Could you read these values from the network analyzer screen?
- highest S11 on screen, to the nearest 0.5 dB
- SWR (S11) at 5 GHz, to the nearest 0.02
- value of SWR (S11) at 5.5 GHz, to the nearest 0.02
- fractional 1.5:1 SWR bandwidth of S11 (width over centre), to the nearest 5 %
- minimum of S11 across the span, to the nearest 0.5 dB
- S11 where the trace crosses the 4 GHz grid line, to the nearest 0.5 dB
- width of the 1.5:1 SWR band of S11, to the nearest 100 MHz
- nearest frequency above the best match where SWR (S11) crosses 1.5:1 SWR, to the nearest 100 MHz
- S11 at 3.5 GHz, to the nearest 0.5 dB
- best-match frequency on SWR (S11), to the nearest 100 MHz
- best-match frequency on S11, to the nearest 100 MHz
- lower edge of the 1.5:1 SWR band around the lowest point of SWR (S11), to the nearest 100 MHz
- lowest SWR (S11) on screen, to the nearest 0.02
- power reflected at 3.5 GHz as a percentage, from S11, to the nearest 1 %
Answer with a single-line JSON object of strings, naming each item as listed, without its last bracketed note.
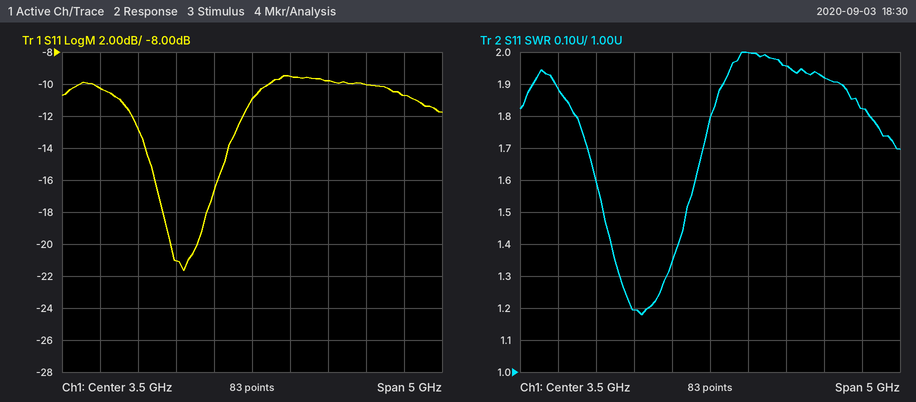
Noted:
{"highest S11 on screen, to the nearest 0.5 dB": "-9.5 dB", "SWR (S11) at 5 GHz, to the nearest 0.02": "1.92", "value of SWR (S11) at 5.5 GHz, to the nearest 0.02": "1.82", "fractional 1.5:1 SWR bandwidth of S11 (width over centre), to the nearest 5 %": "40 %", "minimum of S11 across the span, to the nearest 0.5 dB": "-21.5 dB", "S11 where the trace crosses the 4 GHz grid line, to the nearest 0.5 dB": "-9.5 dB", "width of the 1.5:1 SWR band of S11, to the nearest 100 MHz": "1.1 GHz", "nearest frequency above the best match where SWR (S11) crosses 1.5:1 SWR, to the nearest 100 MHz": "3.2 GHz", "S11 at 3.5 GHz, to the nearest 0.5 dB": "-11.0 dB", "best-match frequency on SWR (S11), to the nearest 100 MHz": "2.6 GHz", "best-match frequency on S11, to the nearest 100 MHz": "2.6 GHz", "lower edge of the 1.5:1 SWR band around the lowest point of SWR (S11), to the nearest 100 MHz": "2.1 GHz", "lowest SWR (S11) on screen, to the nearest 0.02": "1.18", "power reflected at 3.5 GHz as a percentage, from S11, to the nearest 1 %": "8 %"}
